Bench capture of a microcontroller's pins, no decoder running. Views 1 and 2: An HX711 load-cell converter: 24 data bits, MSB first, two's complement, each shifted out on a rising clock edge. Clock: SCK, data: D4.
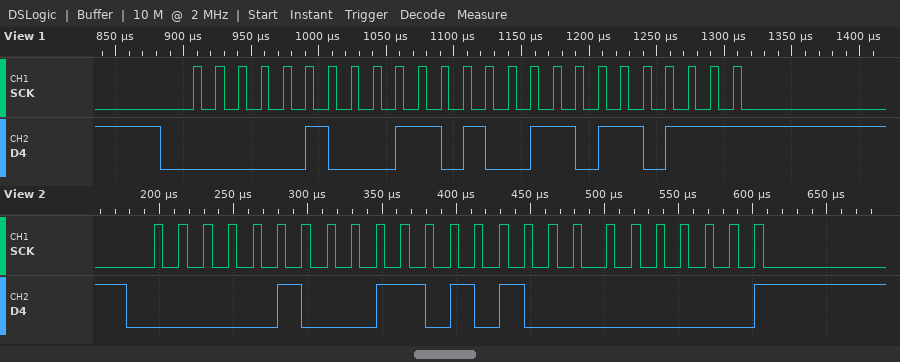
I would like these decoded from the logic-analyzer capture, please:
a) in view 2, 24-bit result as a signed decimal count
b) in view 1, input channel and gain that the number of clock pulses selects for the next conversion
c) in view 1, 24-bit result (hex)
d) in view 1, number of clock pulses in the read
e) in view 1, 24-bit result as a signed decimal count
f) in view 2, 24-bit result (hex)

289280
channel A, gain 128
0x0469B7
25
289207
0x046A00
